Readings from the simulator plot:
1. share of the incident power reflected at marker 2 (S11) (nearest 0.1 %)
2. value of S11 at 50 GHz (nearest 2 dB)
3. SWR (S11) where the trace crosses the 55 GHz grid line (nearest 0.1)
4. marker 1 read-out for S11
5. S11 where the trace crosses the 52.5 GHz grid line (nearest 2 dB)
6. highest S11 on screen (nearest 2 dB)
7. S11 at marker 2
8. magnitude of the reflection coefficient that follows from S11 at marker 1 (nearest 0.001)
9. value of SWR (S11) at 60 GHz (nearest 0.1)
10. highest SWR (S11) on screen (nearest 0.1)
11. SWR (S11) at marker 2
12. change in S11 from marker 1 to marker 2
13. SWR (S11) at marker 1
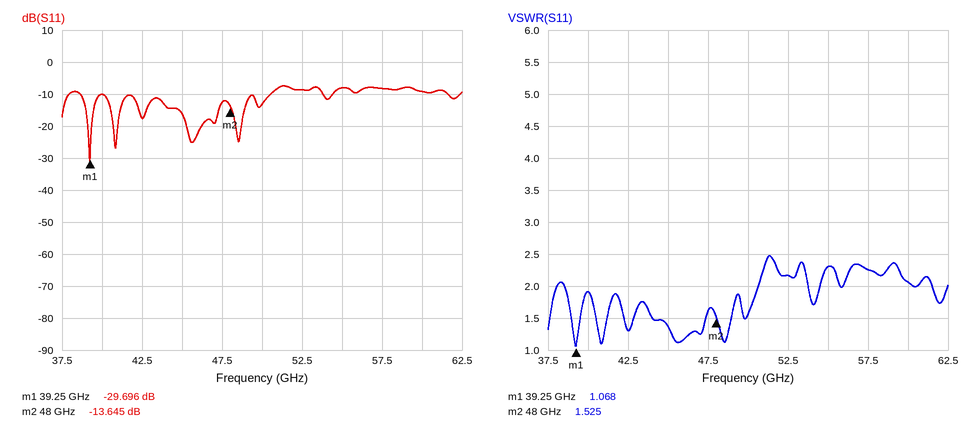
4.3 %
-14 dB
2.3
-29.696 dB
-8 dB
-8 dB
-13.645 dB
0.033
2.1
2.5
1.525
16.051 dB
1.068
